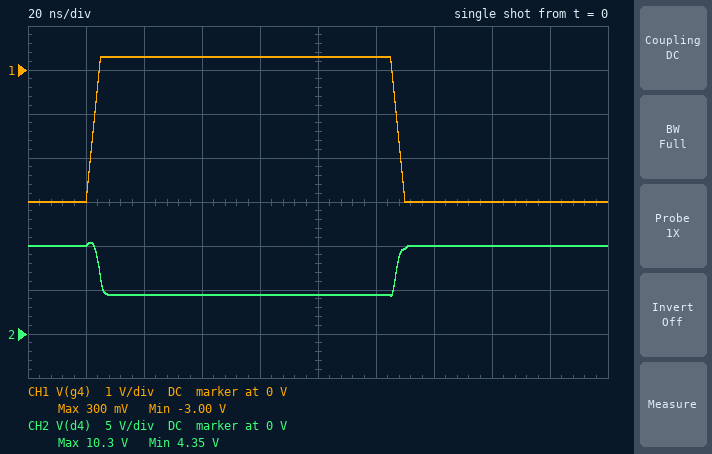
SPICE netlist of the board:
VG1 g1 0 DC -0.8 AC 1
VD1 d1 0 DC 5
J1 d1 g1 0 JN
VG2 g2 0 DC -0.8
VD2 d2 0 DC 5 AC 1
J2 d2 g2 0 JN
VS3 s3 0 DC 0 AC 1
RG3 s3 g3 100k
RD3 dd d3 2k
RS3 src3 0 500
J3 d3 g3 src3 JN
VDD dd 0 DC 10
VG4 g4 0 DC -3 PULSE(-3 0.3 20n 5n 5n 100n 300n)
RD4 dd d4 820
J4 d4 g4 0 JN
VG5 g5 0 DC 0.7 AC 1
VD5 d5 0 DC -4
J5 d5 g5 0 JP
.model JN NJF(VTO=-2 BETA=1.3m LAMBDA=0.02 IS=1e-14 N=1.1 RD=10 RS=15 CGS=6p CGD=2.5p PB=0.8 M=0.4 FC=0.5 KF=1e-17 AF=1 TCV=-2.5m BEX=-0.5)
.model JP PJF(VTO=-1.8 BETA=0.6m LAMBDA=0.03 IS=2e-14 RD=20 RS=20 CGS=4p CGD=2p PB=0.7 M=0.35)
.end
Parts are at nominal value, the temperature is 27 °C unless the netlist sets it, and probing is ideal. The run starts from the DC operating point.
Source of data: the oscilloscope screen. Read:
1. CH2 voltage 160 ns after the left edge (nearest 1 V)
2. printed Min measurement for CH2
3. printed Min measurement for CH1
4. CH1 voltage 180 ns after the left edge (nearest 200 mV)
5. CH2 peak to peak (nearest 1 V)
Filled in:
10 V
4.35 V
-3.00 V
-3.0 V
6 V
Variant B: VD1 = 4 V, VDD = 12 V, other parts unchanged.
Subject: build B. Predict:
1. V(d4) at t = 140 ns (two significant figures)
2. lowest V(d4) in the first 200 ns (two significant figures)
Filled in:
12 V
6.2 V
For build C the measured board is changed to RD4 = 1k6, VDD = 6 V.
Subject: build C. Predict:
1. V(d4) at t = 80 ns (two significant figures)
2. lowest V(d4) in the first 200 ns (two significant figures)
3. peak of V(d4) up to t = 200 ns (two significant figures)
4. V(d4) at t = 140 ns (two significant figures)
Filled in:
730 mV
520 mV
6.6 V
6.0 V
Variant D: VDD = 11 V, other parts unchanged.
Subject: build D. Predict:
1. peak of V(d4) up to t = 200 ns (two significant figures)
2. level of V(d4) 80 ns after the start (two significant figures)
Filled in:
11 V
5.3 V
